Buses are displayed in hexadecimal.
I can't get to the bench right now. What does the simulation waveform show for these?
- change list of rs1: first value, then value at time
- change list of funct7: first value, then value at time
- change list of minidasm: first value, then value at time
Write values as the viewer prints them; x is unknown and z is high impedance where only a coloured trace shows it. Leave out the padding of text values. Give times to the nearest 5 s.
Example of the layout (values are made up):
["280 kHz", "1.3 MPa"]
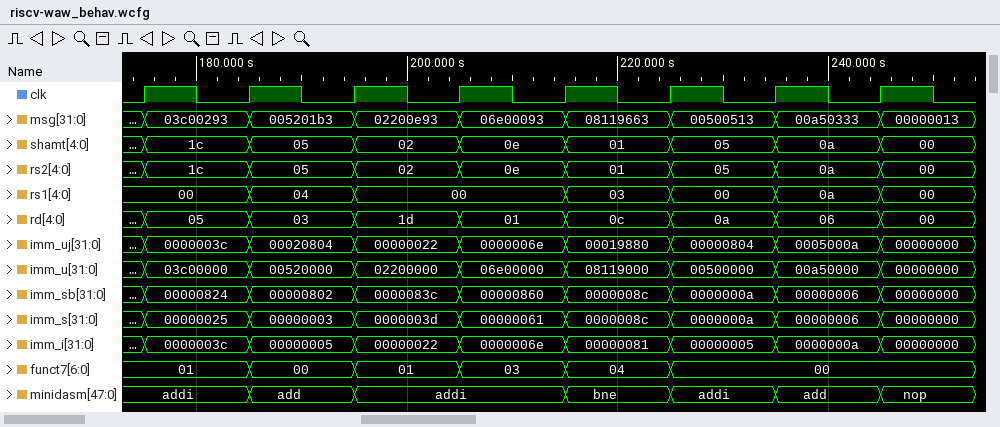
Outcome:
["00, 04 at 185 s, 00 at 195 s, 03 at 215 s, 00 at 225 s, 0a at 235 s, 00 at 245 s", "01, 00 at 185 s, 01 at 195 s, 03 at 205 s, 04 at 215 s, 00 at 225 s", "addi, add at 185 s, addi at 195 s, bne at 215 s, addi at 225 s, add at 235 s, nop at 245 s"]
